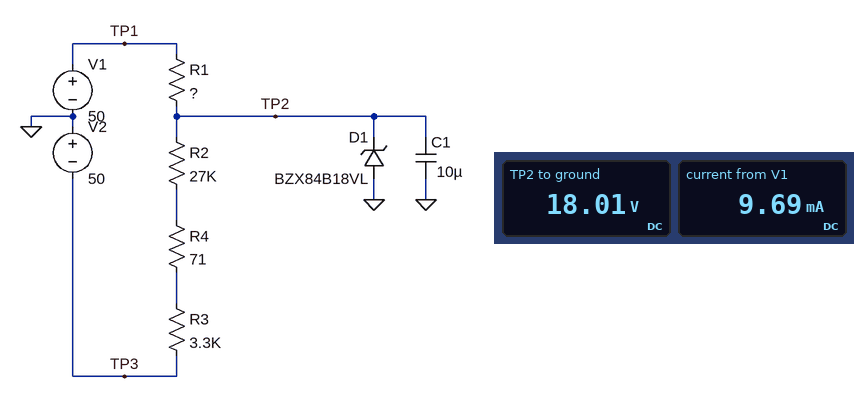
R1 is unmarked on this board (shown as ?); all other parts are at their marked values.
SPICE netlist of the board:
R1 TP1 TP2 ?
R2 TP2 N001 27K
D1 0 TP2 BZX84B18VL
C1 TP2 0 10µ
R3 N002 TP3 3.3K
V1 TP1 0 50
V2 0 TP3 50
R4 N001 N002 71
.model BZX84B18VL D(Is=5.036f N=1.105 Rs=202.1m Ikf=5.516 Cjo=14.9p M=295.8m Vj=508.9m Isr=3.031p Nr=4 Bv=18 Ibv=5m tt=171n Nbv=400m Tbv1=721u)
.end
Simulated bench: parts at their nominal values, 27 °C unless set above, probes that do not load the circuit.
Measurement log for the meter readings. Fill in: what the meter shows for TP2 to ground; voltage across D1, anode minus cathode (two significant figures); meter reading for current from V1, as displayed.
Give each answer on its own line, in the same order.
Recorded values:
18.01 V
-18 V
9.69 mA
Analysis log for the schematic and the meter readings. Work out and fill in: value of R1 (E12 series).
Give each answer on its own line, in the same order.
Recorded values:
3.3 kΩ
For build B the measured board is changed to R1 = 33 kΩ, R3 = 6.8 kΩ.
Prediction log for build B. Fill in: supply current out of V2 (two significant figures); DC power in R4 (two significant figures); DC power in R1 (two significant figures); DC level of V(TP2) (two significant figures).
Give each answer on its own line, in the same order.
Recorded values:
1.5 mA
160 µW
74 mW
650 mV
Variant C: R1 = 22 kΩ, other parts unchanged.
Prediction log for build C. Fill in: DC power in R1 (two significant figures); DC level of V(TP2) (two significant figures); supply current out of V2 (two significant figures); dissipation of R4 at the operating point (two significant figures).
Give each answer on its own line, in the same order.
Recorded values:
80 mW
8.0 V
1.9 mA
260 µW
